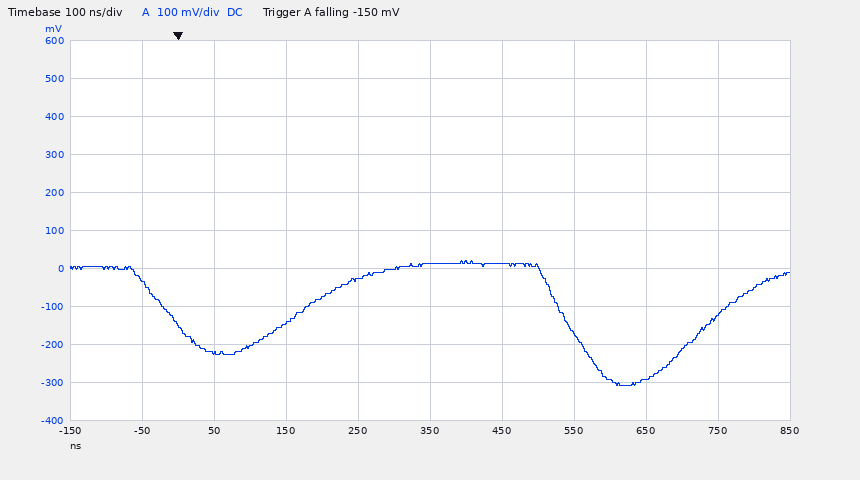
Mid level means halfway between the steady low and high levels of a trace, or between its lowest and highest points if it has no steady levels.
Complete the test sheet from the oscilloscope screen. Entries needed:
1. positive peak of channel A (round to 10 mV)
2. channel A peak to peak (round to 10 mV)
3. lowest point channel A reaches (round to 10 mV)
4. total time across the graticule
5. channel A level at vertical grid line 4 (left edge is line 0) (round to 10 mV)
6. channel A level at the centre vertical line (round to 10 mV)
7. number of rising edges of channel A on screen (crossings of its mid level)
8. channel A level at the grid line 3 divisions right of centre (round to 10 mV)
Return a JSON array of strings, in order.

["20 mV", "330 mV", "-310 mV", "1 µs", "-30 mV", "10 mV", "2", "-290 mV"]
